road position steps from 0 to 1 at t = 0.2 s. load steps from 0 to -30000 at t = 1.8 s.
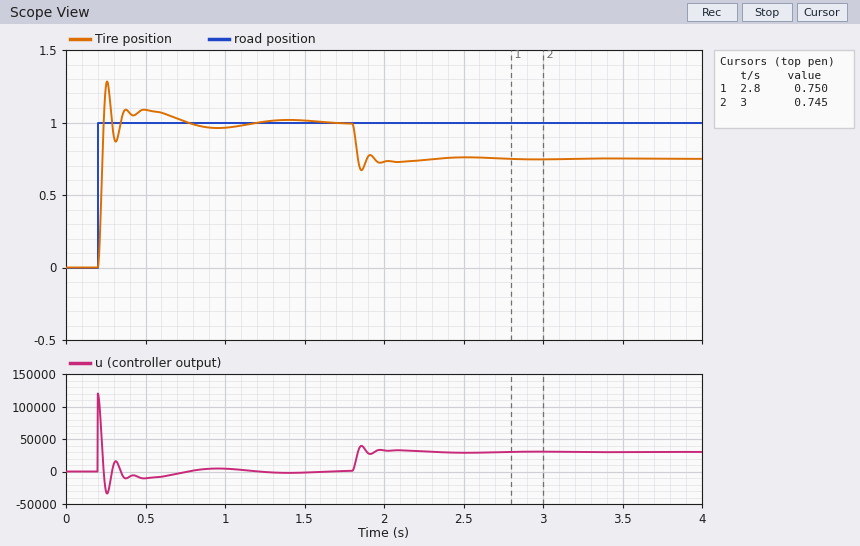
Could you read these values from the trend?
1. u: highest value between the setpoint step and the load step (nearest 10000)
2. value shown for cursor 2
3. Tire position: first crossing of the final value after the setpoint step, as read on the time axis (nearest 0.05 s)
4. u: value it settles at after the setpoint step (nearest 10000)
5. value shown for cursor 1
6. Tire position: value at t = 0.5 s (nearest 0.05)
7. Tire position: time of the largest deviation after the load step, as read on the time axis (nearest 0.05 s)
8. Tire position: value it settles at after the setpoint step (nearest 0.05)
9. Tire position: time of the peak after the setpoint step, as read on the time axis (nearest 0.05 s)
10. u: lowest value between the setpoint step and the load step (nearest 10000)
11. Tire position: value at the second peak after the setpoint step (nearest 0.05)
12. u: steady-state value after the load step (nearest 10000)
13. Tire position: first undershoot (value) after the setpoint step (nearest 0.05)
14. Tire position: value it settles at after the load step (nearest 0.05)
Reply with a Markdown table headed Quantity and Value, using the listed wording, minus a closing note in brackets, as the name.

| Quantity | Value |
|---|---|
| u: highest value between the setpoint step and the load step | 120000 |
| value shown for cursor 2 | 0.745 |
| Tire position: first crossing of the final value after the setpoint step, as read on the time axis | 0.25 s |
| u: value it settles at after the setpoint step | 0 |
| value shown for cursor 1 | 0.750 |
| Tire position: value at t = 0.5 s | 1.10 |
| Tire position: time of the largest deviation after the load step, as read on the time axis | 1.85 s |
| Tire position: value it settles at after the setpoint step | 1.00 |
| Tire position: time of the peak after the setpoint step, as read on the time axis | 0.25 s |
| u: lowest value between the setpoint step and the load step | -30000 |
| Tire position: value at the second peak after the setpoint step | 1.10 |
| u: steady-state value after the load step | 30000 |
| Tire position: first undershoot (value) after the setpoint step | 0.85 |
| Tire position: value it settles at after the load step | 0.75 |
